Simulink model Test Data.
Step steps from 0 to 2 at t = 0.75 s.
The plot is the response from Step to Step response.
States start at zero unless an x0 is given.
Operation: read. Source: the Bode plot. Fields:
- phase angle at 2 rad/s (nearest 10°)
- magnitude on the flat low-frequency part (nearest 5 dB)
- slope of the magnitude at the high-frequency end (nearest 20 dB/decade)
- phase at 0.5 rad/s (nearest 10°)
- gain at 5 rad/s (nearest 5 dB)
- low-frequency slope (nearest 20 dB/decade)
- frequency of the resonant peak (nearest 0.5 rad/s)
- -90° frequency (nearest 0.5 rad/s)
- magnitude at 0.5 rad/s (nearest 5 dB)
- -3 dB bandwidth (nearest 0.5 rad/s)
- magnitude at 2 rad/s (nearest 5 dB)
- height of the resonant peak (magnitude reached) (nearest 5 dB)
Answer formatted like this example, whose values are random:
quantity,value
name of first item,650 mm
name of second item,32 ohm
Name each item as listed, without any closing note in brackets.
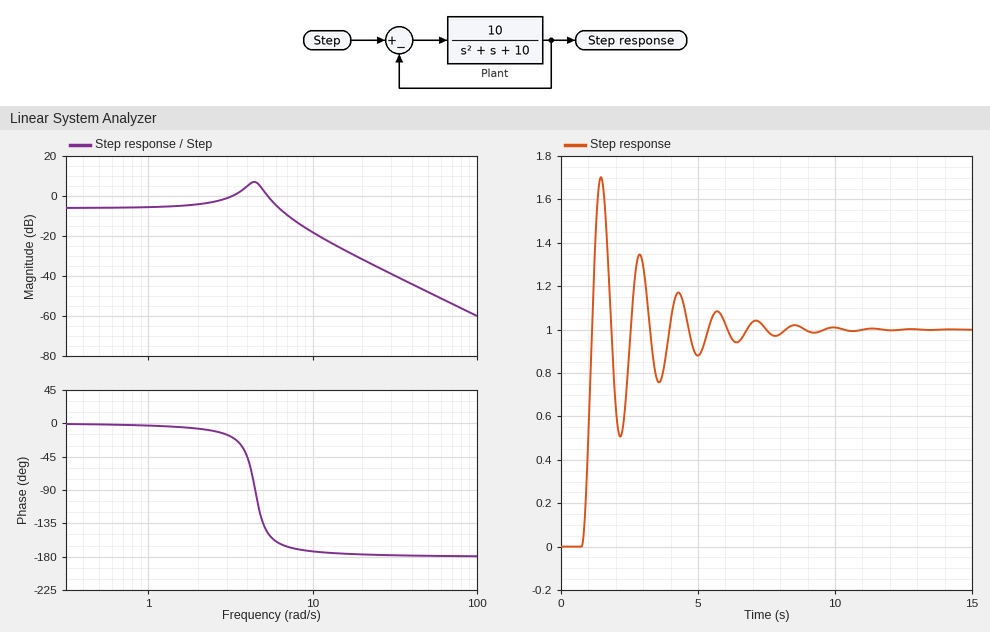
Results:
quantity,value
phase angle at 2 rad/s,-10°
magnitude on the flat low-frequency part,-5 dB
slope of the magnitude at the high-frequency end,-40 dB/decade
phase at 0.5 rad/s,0°
gain at 5 rad/s,5 dB
low-frequency slope,0 dB/decade
frequency of the resonant peak,4.5 rad/s
-90° frequency,4.5 rad/s
magnitude at 0.5 rad/s,-5 dB
-3 dB bandwidth,7.0 rad/s
magnitude at 2 rad/s,-5 dB
height of the resonant peak (magnitude reached),5 dB
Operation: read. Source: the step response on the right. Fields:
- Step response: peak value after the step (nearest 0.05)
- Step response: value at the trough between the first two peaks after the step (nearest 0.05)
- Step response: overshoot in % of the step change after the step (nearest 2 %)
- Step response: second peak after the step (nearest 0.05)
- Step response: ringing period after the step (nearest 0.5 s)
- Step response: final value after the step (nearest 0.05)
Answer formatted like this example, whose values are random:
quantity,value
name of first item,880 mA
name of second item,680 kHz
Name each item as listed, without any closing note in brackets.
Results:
quantity,value
Step response: peak value after the step,1.70
Step response: value at the trough between the first two peaks after the step,0.50
Step response: overshoot in % of the step change after the step,70 %
Step response: second peak after the step,1.35
Step response: ringing period after the step,1.5 s
Step response: final value after the step,1.00
